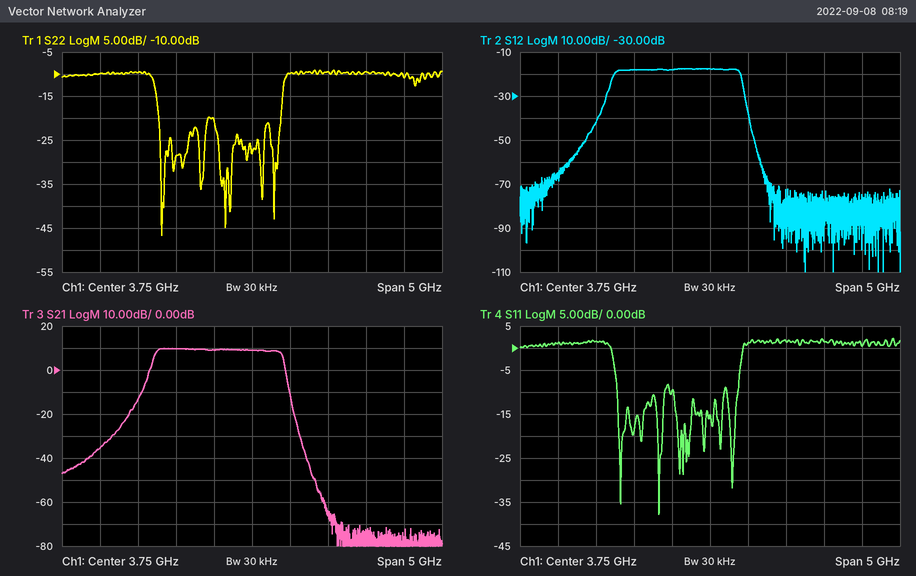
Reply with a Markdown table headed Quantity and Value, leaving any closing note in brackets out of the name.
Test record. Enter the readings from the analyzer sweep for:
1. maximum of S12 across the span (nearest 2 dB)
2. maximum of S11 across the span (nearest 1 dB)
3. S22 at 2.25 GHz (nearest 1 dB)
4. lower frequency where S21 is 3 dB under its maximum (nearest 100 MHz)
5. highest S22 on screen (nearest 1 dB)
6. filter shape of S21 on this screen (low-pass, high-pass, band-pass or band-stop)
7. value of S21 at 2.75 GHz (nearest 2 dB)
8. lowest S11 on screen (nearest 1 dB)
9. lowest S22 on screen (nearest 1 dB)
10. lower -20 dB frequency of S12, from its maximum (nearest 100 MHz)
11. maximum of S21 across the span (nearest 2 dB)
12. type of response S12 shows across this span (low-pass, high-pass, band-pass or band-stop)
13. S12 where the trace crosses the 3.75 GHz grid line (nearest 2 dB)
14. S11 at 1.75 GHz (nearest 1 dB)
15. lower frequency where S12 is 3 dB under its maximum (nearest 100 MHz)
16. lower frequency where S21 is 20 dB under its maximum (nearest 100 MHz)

| Quantity | Value |
|---|---|
| maximum of S12 across the span | -18 dB |
| maximum of S11 across the span | 2 dB |
| S22 at 2.25 GHz | -10 dB |
| lower frequency where S21 is 3 dB under its maximum | 2.5 GHz |
| highest S22 on screen | -9 dB |
| filter shape of S21 on this screen | band-pass |
| value of S21 at 2.75 GHz | 10 dB |
| lowest S11 on screen | -38 dB |
| lowest S22 on screen | -47 dB |
| lower -20 dB frequency of S12, from its maximum | 2.3 GHz |
| maximum of S21 across the span | 10 dB |
| type of response S12 shows across this span | band-pass |
| S12 where the trace crosses the 3.75 GHz grid line | -18 dB |
| S11 at 1.75 GHz | 1 dB |
| lower frequency where S12 is 3 dB under its maximum | 2.5 GHz |
| lower frequency where S21 is 20 dB under its maximum | 2.3 GHz |
